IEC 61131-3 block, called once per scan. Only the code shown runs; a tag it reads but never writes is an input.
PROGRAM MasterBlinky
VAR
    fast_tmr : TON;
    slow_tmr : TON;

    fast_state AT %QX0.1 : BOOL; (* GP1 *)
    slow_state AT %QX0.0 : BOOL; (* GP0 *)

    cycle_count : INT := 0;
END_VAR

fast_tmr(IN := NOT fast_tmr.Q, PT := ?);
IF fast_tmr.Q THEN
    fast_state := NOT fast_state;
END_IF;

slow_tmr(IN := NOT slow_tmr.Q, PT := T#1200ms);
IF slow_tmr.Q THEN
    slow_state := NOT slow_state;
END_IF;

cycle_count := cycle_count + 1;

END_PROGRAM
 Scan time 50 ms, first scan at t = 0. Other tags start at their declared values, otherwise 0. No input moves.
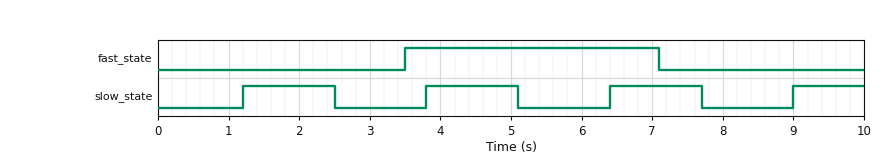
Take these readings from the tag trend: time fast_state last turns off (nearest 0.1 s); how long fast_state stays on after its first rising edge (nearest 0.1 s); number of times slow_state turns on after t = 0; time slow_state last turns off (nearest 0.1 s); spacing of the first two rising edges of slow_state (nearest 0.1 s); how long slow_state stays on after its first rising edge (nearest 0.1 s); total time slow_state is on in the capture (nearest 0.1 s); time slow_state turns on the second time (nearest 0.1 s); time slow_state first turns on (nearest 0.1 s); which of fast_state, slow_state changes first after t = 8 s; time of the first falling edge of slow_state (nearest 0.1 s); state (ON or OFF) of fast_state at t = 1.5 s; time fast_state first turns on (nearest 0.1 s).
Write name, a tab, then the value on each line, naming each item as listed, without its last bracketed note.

time fast_state last turns off	7.1 s
how long fast_state stays on after its first rising edge	3.6 s
number of times slow_state turns on after t = 0	4
time slow_state last turns off	7.7 s
spacing of the first two rising edges of slow_state	2.6 s
how long slow_state stays on after its first rising edge	1.3 s
total time slow_state is on in the capture	4.9 s
time slow_state turns on the second time	3.8 s
time slow_state first turns on	1.2 s
which of fast_state, slow_state changes first after t = 8 s	slow_state
time of the first falling edge of slow_state	2.5 s
state (ON or OFF) of fast_state at t = 1.5 s	OFF
time fast_state first turns on	3.5 s
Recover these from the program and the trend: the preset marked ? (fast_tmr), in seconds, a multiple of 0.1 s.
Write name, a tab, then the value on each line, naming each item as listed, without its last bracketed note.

the preset marked ? (fast_tmr), in seconds, a multiple of 0.1 s	3.5 s
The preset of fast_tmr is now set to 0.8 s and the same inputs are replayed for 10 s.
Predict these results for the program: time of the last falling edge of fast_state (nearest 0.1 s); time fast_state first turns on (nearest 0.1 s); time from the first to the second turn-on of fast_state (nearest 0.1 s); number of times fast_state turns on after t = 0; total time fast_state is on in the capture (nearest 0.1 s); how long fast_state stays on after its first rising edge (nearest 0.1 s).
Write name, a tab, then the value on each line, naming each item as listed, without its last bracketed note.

time of the last falling edge of fast_state	8.9 s
time fast_state first turns on	0.8 s
time from the first to the second turn-on of fast_state	1.8 s
number of times fast_state turns on after t = 0	6
total time fast_state is on in the capture	4.7 s
how long fast_state stays on after its first rising edge	0.9 s
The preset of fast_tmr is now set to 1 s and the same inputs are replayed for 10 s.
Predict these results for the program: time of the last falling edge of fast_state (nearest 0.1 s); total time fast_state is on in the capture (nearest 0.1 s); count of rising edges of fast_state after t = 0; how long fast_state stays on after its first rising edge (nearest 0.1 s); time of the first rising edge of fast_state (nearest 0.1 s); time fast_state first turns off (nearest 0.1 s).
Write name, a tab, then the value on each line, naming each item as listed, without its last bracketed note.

time of the last falling edge of fast_state	8.7 s
total time fast_state is on in the capture	4.6 s
count of rising edges of fast_state after t = 0	5
how long fast_state stays on after its first rising edge	1.1 s
time of the first rising edge of fast_state	1.0 s
time fast_state first turns off	2.1 s
